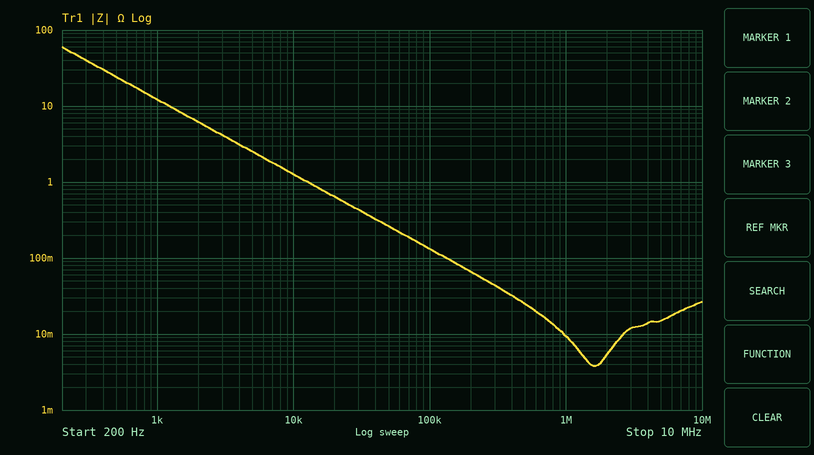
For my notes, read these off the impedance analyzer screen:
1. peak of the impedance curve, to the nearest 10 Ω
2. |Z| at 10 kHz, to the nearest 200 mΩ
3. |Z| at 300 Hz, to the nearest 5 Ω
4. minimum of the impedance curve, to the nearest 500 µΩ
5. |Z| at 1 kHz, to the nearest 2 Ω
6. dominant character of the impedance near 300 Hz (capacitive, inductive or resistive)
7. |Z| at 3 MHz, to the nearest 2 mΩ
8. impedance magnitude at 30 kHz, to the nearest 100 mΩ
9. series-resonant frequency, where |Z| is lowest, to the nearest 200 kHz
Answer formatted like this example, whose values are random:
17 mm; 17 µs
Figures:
60 Ω; 1.2 Ω; 40 Ω; 4.0 mΩ; 12 Ω; capacitive; 12 mΩ; 400 mΩ; 1.6 MHz
